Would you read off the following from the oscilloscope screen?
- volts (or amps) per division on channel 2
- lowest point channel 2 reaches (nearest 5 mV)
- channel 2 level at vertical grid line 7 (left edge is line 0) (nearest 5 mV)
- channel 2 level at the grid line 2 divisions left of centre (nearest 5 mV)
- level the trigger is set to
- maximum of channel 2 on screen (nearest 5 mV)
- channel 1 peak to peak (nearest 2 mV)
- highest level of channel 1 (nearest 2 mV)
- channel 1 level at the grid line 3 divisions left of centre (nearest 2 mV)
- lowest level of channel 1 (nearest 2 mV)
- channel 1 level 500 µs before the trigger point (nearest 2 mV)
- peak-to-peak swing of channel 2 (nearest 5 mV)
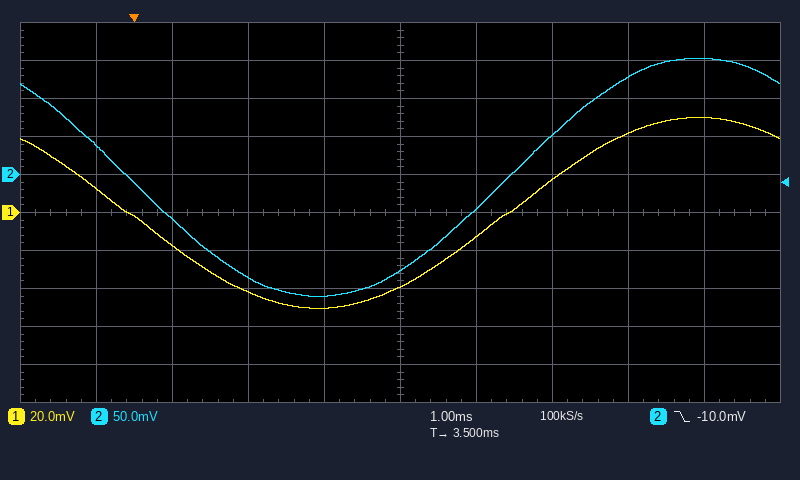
50 mV
-160 mV
50 mV
-135 mV
-10.0 mV
155 mV
100 mV
50 mV
-18 mV
-50 mV
12 mV
315 mV
